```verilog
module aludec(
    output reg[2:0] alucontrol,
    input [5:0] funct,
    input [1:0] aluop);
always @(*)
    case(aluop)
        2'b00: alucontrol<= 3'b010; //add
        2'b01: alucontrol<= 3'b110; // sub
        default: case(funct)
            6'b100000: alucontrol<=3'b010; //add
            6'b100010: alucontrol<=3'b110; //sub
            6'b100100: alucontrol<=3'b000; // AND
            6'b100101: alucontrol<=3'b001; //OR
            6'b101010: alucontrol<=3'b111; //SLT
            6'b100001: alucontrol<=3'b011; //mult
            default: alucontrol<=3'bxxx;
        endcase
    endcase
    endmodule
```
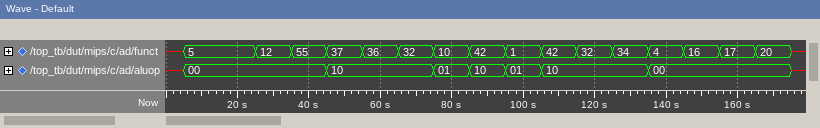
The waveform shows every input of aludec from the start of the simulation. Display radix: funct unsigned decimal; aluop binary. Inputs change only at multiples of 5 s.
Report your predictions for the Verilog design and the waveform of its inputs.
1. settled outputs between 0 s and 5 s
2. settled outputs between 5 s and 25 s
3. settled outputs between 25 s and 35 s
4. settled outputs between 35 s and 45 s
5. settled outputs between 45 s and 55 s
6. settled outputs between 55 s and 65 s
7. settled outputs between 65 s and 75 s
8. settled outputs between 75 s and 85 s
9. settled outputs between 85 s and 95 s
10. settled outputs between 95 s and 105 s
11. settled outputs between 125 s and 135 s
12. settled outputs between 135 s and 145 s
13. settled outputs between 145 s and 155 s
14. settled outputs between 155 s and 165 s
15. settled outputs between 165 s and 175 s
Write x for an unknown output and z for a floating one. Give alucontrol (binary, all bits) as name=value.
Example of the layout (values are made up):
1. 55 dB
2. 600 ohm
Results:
1. alucontrol=x
2. alucontrol=010
3. alucontrol=010
4. alucontrol=010
5. alucontrol=001
6. alucontrol=000
7. alucontrol=010
8. alucontrol=110
9. alucontrol=111
10. alucontrol=110
11. alucontrol=110
12. alucontrol=010
13. alucontrol=010
14. alucontrol=010
15. alucontrol=010
